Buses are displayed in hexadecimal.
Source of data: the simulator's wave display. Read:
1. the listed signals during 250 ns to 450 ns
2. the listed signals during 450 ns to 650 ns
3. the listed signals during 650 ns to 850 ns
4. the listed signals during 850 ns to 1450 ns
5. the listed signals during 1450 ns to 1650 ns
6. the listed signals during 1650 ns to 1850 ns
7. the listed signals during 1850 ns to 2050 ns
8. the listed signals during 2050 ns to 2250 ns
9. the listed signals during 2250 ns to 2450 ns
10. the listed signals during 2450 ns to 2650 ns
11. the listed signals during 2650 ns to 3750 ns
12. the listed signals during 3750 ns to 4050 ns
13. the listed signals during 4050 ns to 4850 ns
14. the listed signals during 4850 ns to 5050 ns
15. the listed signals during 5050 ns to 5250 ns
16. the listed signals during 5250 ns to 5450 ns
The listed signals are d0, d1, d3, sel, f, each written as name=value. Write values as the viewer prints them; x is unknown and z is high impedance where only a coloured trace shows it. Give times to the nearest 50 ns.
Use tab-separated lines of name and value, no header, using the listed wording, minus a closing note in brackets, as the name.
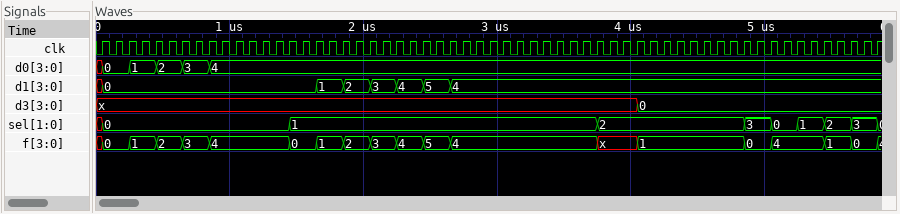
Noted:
the listed signals during 250 ns to 450 ns	d0=1, d1=0, d3=x, sel=0, f=1
the listed signals during 450 ns to 650 ns	d0=2, d1=0, d3=x, sel=0, f=2
the listed signals during 650 ns to 850 ns	d0=3, d1=0, d3=x, sel=0, f=3
the listed signals during 850 ns to 1450 ns	d0=4, d1=0, d3=x, sel=0, f=4
the listed signals during 1450 ns to 1650 ns	d0=4, d1=0, d3=x, sel=1, f=0
the listed signals during 1650 ns to 1850 ns	d0=4, d1=1, d3=x, sel=1, f=1
the listed signals during 1850 ns to 2050 ns	d0=4, d1=2, d3=x, sel=1, f=2
the listed signals during 2050 ns to 2250 ns	d0=4, d1=3, d3=x, sel=1, f=3
the listed signals during 2250 ns to 2450 ns	d0=4, d1=4, d3=x, sel=1, f=4
the listed signals during 2450 ns to 2650 ns	d0=4, d1=5, d3=x, sel=1, f=5
the listed signals during 2650 ns to 3750 ns	d0=4, d1=4, d3=x, sel=1, f=4
the listed signals during 3750 ns to 4050 ns	d0=4, d1=4, d3=x, sel=2, f=x
the listed signals during 4050 ns to 4850 ns	d0=4, d1=4, d3=0, sel=2, f=1
the listed signals during 4850 ns to 5050 ns	d0=4, d1=4, d3=0, sel=3, f=0
the listed signals during 5050 ns to 5250 ns	d0=4, d1=4, d3=0, sel=0, f=4
the listed signals during 5250 ns to 5450 ns	d0=4, d1=4, d3=0, sel=1, f=4
